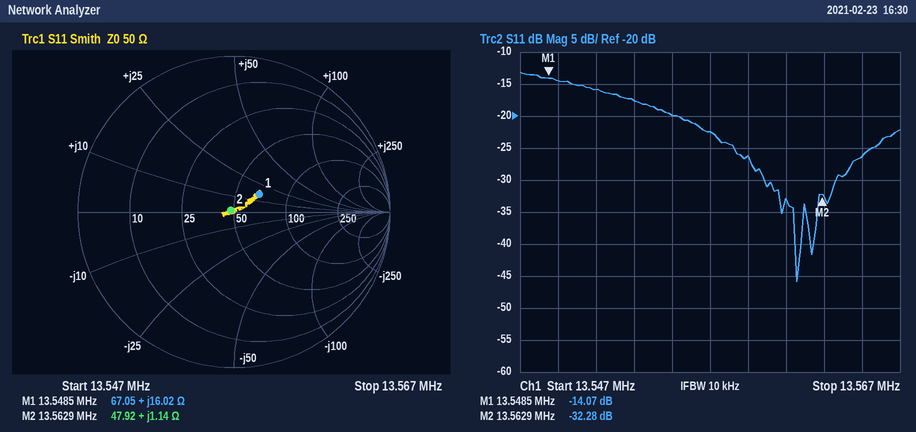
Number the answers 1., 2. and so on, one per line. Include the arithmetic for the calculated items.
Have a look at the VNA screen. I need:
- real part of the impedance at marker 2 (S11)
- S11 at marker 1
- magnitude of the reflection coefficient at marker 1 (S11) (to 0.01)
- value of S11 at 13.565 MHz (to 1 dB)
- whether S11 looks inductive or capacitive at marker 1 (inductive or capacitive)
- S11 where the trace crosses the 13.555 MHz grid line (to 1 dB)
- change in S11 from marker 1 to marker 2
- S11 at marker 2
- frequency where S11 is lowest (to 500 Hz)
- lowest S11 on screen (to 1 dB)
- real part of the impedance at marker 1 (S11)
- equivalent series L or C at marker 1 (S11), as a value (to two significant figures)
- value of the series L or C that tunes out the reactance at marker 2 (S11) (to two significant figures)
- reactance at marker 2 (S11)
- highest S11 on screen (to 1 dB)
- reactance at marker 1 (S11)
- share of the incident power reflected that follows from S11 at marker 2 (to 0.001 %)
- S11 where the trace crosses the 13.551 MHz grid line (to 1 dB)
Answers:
1. 47.92 Ω
2. -14.07 dB
3. 0.20
4. -26 dB
5. inductive
6. -20 dB
7. -32.28 − (-14.07) = -18.21 dB
8. -32.28 dB
9. 13.5615 MHz
10. -46 dB
11. 67.05 Ω
12. L = 16.02 Ω/(2π × 13.5485 MHz) ≈ 188 nH, so 190 nH to two significant figures
13. C = 1/(2π × 13.5629 MHz × 1.14 Ω) ≈ 10 nF
14. +1.14 Ω
15. -13 dB
16. +16.02 Ω
17. 10^(-32.28/10) ≈ 0.059 %
18. -16 dB
